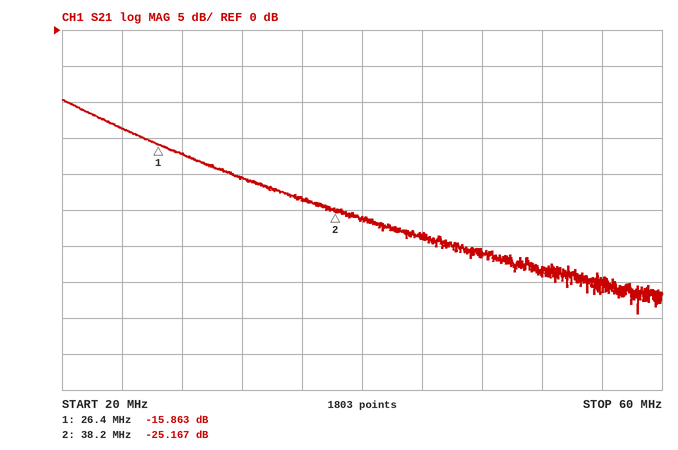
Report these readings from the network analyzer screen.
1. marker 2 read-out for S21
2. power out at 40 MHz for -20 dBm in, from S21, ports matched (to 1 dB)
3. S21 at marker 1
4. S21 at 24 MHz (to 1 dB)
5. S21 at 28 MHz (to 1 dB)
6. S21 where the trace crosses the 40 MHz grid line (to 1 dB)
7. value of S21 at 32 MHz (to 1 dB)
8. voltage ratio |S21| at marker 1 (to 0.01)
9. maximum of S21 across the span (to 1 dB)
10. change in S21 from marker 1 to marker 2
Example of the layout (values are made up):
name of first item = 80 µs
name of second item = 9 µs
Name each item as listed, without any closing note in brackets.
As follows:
marker 2 read-out for S21 = -25.167 dB
power out at 40 MHz for -20 dBm in, from S21, ports matched = -46 dBm
S21 at marker 1 = -15.863 dB
S21 at 24 MHz = -14 dB
S21 at 28 MHz = -17 dB
S21 where the trace crosses the 40 MHz grid line = -26 dB
value of S21 at 32 MHz = -20 dB
voltage ratio |S21| at marker 1 = 0.16
maximum of S21 across the span = -10 dB
change in S21 from marker 1 to marker 2 = -9.304 dB
